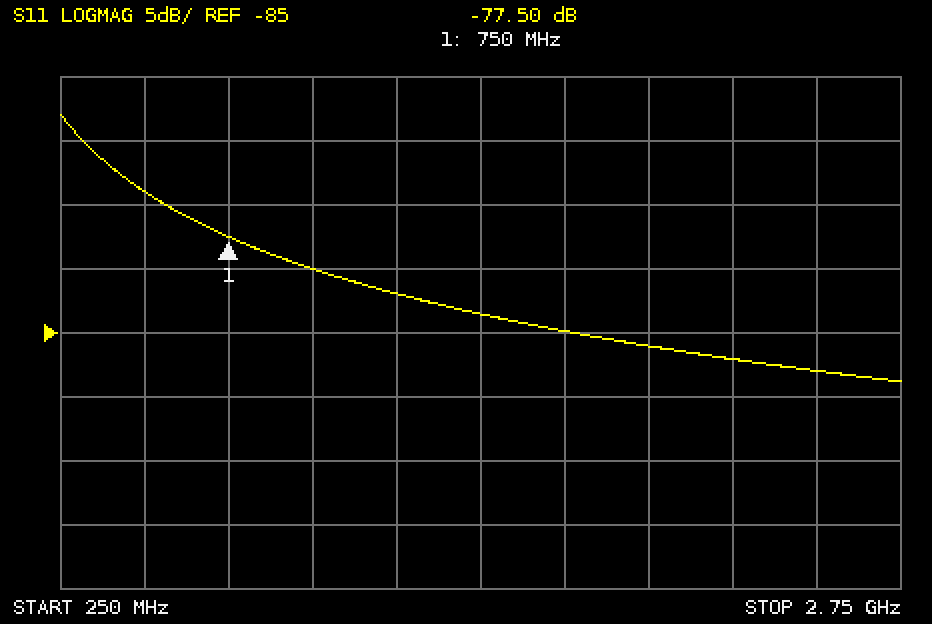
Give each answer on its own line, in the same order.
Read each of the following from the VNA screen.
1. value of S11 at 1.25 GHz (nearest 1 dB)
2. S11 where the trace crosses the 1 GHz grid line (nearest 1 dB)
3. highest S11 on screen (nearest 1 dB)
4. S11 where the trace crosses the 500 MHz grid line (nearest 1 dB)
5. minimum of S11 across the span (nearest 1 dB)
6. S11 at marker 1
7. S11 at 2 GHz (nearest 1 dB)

-82 dB
-80 dB
-68 dB
-74 dB
-89 dB
-77.50 dB
-86 dB
